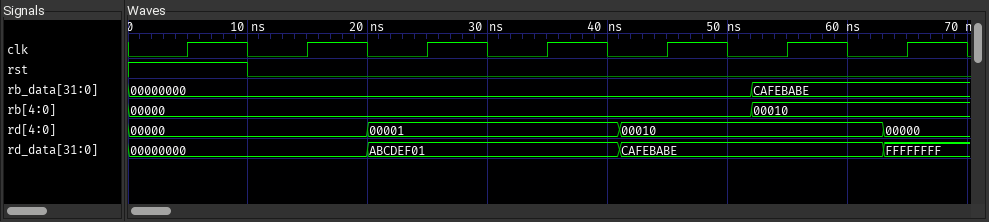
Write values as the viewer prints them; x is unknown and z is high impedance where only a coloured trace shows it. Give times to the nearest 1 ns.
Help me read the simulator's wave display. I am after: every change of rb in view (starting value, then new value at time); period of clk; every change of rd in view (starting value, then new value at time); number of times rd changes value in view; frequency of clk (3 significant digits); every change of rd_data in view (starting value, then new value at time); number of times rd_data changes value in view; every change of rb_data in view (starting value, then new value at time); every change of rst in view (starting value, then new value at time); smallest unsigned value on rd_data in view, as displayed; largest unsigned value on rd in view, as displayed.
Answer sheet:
00000, 00010 at 52 ns
10 ns
00000, 00001 at 20 ns, 00010 at 41 ns, 00000 at 63 ns
3
100 MHz
00000000, ABCDEF01 at 20 ns, CAFEBABE at 41 ns, FFFFFFFF at 63 ns
3
00000000, CAFEBABE at 52 ns
1, 0 at 10 ns
00000000
00010
